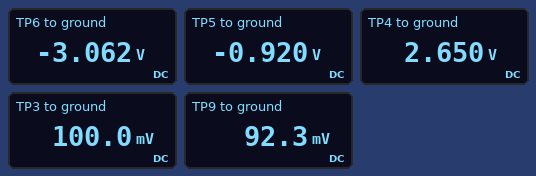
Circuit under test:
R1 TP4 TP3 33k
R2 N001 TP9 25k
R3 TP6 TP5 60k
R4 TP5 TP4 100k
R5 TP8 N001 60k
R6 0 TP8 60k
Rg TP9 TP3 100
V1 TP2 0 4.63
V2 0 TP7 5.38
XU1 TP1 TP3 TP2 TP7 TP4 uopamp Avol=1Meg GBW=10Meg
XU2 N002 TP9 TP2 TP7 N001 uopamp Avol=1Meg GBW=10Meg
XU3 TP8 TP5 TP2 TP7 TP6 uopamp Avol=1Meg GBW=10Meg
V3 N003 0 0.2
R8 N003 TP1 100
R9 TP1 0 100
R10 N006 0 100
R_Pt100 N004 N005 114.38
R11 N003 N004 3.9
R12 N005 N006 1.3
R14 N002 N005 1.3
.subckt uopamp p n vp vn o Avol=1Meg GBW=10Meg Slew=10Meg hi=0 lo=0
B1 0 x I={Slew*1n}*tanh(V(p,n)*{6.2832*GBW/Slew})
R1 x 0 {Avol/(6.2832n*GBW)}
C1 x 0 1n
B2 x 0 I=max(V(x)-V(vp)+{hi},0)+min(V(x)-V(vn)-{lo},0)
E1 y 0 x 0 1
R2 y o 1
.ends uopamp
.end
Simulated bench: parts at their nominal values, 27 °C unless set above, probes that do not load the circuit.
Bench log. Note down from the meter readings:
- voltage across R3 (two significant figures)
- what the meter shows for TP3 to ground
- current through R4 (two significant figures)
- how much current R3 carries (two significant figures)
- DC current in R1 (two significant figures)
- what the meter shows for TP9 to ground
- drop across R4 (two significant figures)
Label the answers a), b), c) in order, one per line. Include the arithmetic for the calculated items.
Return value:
a) -920 mV - (-3.062 V) = 2.1 V
b) 100.0 mV
c) (2.65 V - (-920 mV)) / 100 kΩ = 36 µA
d) (-920 mV - (-3.062 V)) / 60 kΩ = 36 µA
e) (2.65 V - 100 mV) / 33 kΩ = 77 µA
f) 92.3 mV
g) 2.65 V - (-920 mV) = 3.6 V
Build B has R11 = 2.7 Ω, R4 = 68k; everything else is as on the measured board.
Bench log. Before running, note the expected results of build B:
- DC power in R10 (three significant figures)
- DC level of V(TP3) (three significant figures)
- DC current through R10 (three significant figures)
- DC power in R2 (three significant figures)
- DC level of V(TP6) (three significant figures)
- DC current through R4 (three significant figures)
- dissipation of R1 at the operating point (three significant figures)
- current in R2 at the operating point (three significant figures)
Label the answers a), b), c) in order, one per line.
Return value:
a) 83.9 µW
b) 100 mV
c) 916 µA
d) 130 µW
e) -3.80 V
f) 49.1 µA
g) 172 µW
h) 72.2 µA
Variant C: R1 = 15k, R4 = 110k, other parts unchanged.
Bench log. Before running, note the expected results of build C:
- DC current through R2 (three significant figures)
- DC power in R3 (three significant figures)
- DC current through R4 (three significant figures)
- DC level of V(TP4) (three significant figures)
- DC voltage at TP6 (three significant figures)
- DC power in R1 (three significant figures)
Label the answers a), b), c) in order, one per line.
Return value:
a) 77.3 µA
b) 23.6 µW
c) 19.8 µA
d) 1.26 V
e) -2.11 V
f) 89.6 µW
